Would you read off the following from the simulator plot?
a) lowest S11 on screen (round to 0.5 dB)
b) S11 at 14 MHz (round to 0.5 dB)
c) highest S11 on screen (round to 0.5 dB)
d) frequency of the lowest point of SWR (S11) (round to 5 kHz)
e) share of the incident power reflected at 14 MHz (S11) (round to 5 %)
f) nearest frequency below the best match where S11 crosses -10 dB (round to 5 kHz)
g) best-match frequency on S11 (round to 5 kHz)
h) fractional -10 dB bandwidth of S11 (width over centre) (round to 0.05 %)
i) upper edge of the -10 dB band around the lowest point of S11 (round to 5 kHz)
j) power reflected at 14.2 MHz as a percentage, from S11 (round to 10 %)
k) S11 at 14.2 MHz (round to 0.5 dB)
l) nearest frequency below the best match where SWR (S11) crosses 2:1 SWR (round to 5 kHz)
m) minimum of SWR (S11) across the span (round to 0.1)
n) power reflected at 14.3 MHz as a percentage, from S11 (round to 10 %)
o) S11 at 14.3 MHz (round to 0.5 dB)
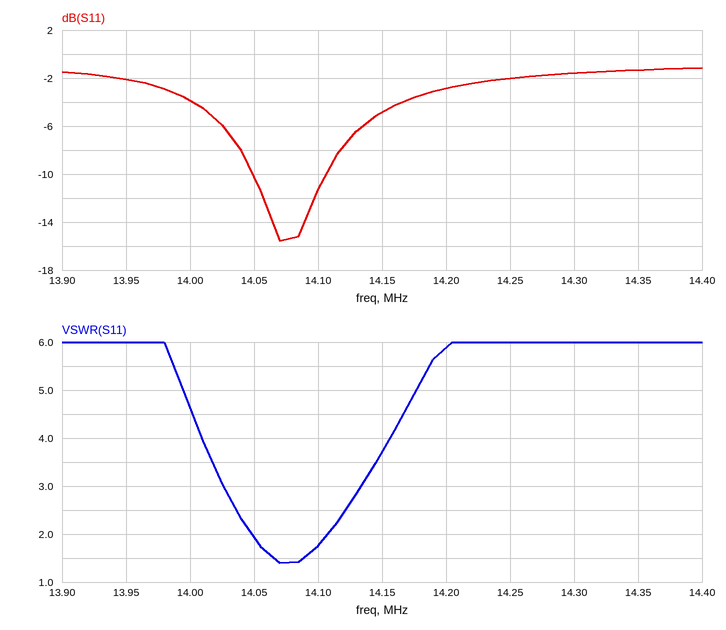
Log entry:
-15.5 dB
-4.0 dB
-1.0 dB
14.070 MHz
40 %
14.050 MHz
14.070 MHz
0.40 %
14.105 MHz
50 %
-3.0 dB
14.050 MHz
1.4
70 %
-1.5 dB
